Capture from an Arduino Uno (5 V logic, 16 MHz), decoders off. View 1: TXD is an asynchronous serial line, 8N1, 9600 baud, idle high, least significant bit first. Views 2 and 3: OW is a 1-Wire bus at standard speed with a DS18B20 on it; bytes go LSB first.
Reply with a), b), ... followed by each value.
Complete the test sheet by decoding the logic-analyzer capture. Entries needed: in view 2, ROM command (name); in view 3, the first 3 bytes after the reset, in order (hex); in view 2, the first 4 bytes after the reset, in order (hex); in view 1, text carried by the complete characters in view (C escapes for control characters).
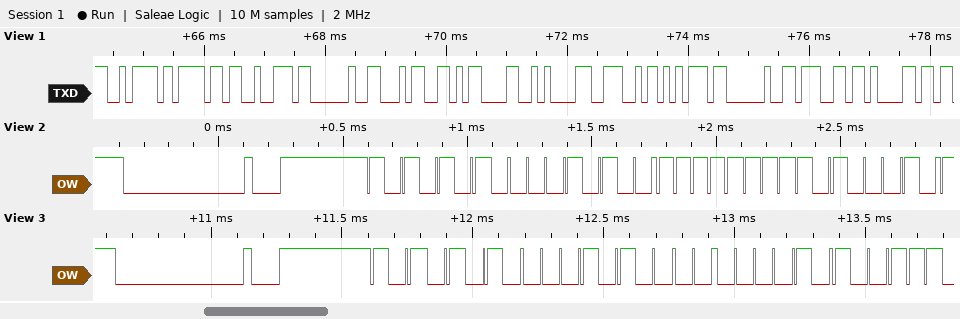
a) Match ROM
b) 55 28 40
c) 55 28 FF 45
d) "zor 4\r\nNu ga"
